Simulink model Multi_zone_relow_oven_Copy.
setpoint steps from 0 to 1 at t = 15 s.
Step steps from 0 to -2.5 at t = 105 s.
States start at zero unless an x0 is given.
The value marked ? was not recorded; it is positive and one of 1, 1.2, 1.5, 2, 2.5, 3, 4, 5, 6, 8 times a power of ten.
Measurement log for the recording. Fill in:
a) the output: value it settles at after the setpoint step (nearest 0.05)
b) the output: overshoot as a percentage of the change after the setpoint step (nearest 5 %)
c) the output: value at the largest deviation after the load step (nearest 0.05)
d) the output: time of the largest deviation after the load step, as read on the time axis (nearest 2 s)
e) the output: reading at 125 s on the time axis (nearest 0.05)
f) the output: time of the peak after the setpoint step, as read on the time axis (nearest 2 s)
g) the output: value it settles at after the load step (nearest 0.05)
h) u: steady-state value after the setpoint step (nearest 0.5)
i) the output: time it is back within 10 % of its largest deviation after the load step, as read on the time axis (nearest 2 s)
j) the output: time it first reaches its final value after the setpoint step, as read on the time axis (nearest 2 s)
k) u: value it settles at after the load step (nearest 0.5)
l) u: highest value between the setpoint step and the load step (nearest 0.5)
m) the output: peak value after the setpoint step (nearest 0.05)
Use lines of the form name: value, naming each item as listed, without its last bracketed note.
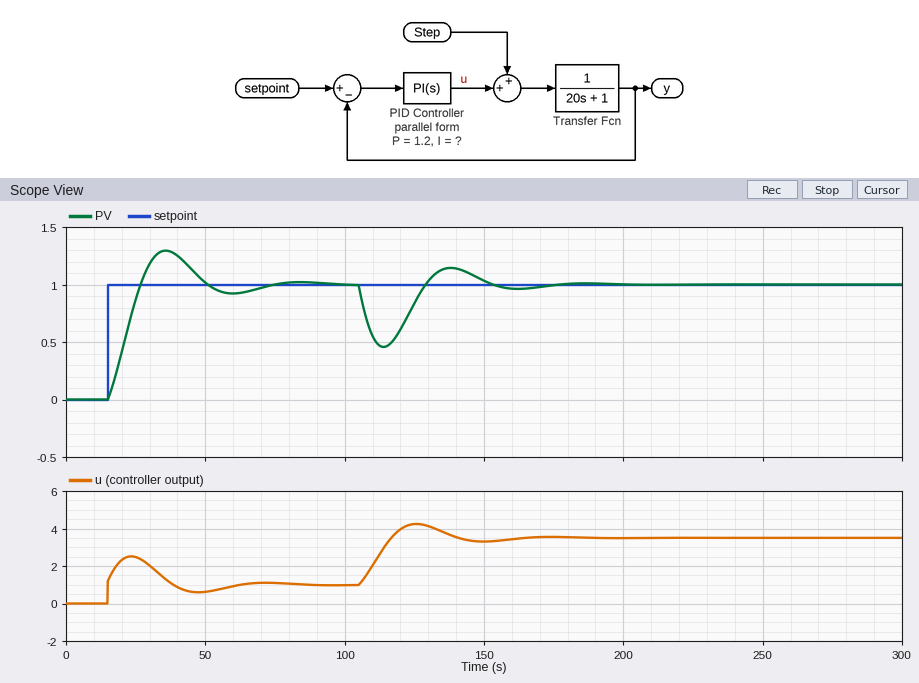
the output: value it settles at after the setpoint step: 1.00
the output: overshoot as a percentage of the change after the setpoint step: 30 %
the output: value at the largest deviation after the load step: 0.45
the output: time of the largest deviation after the load step, as read on the time axis: 114 s
the output: reading at 125 s on the time axis: 0.85
the output: time of the peak after the setpoint step, as read on the time axis: 36 s
the output: value it settles at after the load step: 1.00
u: steady-state value after the setpoint step: 1.0
the output: time it is back within 10 % of its largest deviation after the load step, as read on the time axis: 148 s
the output: time it first reaches its final value after the setpoint step, as read on the time axis: 26 s
u: value it settles at after the load step: 3.5
u: highest value between the setpoint step and the load step: 2.5
the output: peak value after the setpoint step: 1.30
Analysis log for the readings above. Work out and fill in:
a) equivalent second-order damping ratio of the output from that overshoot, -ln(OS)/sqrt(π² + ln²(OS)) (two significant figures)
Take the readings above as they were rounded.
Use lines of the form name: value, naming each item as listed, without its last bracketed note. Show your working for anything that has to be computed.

equivalent second-order damping ratio of the output from that overshoot, -ln(OS)/sqrt(π² + ln²(OS)): ln(0.3) = -1.204; 1.204 / sqrt(9.870 + 1.450) = 0.36
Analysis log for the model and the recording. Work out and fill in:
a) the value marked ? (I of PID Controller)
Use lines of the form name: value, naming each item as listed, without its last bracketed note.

the value marked ?: 0.4
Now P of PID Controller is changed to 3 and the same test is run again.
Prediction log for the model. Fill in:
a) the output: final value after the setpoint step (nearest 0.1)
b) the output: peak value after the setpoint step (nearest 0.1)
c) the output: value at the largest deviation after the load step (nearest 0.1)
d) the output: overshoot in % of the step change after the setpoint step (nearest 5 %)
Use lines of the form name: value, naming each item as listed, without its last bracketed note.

the output: final value after the setpoint step: 1.0
the output: peak value after the setpoint step: 1.1
the output: value at the largest deviation after the load step: 0.6
the output: overshoot in % of the step change after the setpoint step: 10 %
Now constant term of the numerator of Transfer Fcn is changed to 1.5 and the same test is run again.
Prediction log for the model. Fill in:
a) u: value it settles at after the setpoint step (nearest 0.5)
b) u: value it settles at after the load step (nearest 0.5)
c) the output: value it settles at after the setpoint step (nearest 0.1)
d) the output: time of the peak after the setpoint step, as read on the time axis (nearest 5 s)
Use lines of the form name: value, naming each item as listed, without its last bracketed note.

u: value it settles at after the setpoint step: 0.5
u: value it settles at after the load step: 3.0
the output: value it settles at after the setpoint step: 1.0
the output: time of the peak after the setpoint step, as read on the time axis: 30 s
